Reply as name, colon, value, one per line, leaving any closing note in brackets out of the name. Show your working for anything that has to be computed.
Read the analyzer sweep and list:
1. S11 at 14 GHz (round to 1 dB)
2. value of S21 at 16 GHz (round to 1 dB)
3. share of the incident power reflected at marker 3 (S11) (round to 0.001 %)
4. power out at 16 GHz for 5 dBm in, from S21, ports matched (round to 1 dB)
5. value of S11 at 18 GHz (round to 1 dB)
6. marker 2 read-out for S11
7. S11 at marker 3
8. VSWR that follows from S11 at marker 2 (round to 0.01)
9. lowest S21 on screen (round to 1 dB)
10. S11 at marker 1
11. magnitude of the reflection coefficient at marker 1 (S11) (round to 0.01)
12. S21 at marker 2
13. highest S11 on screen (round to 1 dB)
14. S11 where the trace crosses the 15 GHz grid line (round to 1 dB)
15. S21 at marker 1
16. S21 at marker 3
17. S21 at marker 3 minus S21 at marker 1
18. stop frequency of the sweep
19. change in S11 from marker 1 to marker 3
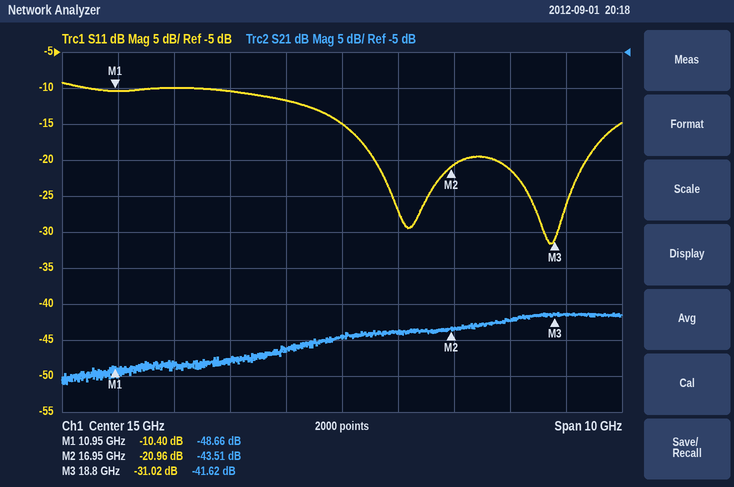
S11 at 14 GHz: -12 dB
value of S21 at 16 GHz: -44 dB
share of the incident power reflected at marker 3 (S11): 10^(-31.02/10) ≈ 0.079 %
power out at 16 GHz for 5 dBm in, from S21, ports matched: 5 dBm + (-44 dB) = -39 dBm
value of S11 at 18 GHz: -21 dB
marker 2 read-out for S11: -20.96 dB
S11 at marker 3: -31.02 dB
VSWR that follows from S11 at marker 2: (1 + 0.0895)/(1 − 0.0895) ≈ 1.20
lowest S21 on screen: -51 dB
S11 at marker 1: -10.40 dB
magnitude of the reflection coefficient at marker 1 (S11): 10^(-10.4/20) ≈ 0.30
S21 at marker 2: -43.51 dB
highest S11 on screen: -9 dB
S11 where the trace crosses the 15 GHz grid line: -15 dB
S21 at marker 1: -48.66 dB
S21 at marker 3: -41.62 dB
S21 at marker 3 minus S21 at marker 1: -41.62 − (-48.66) = 7.04 dB
stop frequency of the sweep: 20 GHz
change in S11 from marker 1 to marker 3: -31.02 − (-10.4) = -20.62 dB
